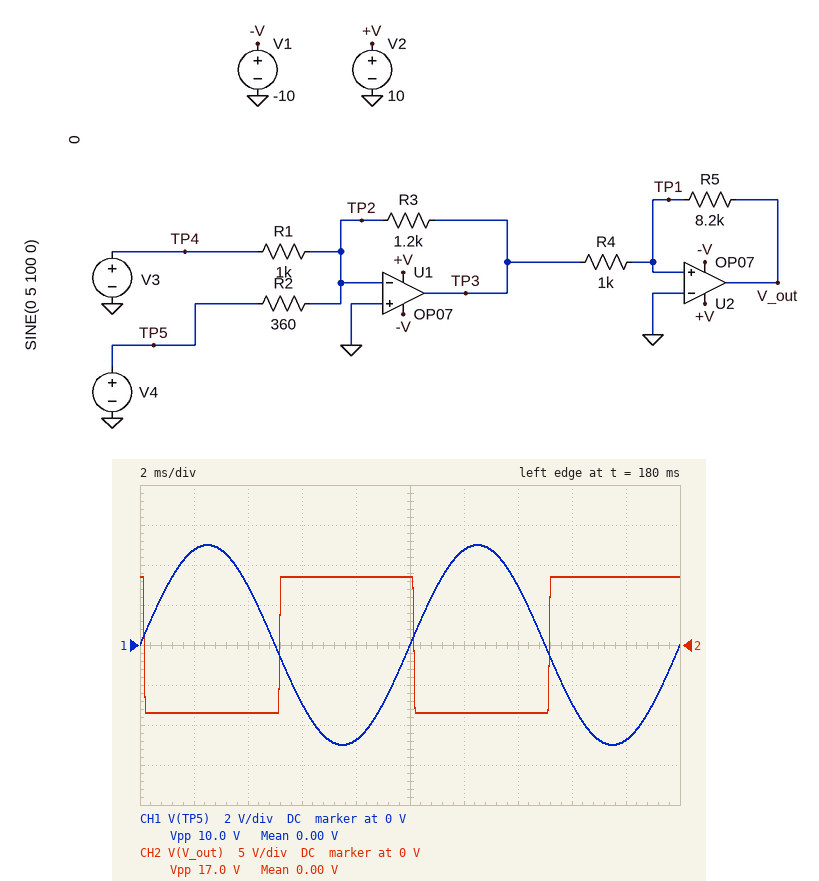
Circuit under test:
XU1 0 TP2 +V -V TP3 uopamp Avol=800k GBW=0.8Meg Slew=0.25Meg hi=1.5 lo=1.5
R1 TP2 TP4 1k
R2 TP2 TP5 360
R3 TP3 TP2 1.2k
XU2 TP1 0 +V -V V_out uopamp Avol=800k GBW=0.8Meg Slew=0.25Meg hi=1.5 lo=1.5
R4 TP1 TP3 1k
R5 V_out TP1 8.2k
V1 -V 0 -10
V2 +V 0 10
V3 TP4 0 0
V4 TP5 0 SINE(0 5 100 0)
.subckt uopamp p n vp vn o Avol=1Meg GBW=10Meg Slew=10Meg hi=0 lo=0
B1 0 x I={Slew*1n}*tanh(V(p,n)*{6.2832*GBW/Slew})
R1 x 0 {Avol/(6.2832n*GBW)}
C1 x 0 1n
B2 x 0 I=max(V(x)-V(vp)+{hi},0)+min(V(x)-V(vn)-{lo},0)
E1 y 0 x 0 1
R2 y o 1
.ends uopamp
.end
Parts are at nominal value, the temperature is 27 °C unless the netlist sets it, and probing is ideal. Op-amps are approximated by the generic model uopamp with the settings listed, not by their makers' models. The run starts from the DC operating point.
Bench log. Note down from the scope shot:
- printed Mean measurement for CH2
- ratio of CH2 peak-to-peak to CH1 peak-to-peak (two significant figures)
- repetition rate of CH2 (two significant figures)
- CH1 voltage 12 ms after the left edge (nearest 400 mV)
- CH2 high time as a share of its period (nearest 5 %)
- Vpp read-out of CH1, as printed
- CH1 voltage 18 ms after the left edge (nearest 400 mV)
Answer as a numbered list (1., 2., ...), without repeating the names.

1. 0.00 V
2. 1.7
3. 100 Hz
4. 4.8 V
5. 50 %
6. 10.0 V
7. -4.8 V
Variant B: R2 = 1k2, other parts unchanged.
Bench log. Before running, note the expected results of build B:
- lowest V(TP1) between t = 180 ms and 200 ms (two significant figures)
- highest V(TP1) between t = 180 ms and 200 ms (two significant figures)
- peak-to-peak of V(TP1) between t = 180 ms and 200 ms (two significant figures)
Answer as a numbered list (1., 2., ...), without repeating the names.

1. -5.4 V
2. 5.4 V
3. 11 V
